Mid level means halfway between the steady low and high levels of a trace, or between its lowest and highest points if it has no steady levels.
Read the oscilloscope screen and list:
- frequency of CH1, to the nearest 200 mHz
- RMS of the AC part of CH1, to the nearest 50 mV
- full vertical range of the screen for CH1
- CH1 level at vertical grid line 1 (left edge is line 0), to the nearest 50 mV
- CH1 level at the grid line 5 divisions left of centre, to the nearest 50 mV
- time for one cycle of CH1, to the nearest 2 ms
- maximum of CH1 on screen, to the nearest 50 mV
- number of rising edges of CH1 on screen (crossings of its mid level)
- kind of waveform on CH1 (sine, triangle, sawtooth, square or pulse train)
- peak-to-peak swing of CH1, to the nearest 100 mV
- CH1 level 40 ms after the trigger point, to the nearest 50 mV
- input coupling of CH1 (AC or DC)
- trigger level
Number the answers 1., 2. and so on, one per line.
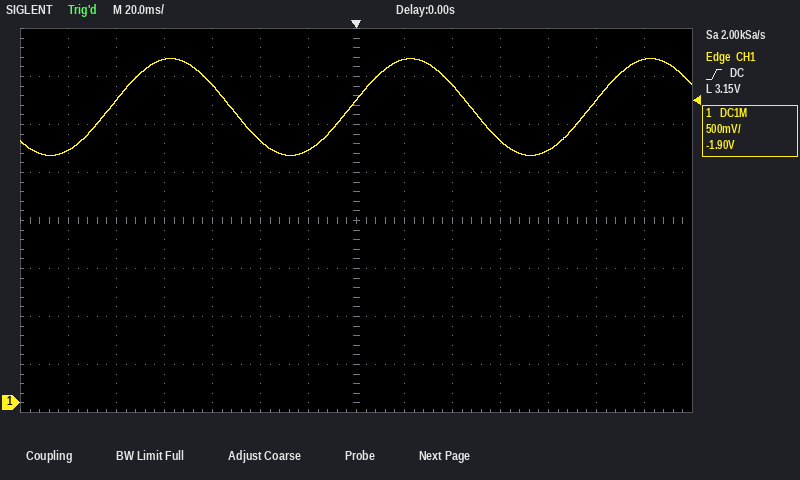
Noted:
1. 10.0 Hz
2. 350 mV
3. 4 V
4. 2.65 V
5. 3.15 V
6. 100 ms
7. 3.60 V
8. 3
9. sine
10. 1.00 V
11. 3.30 V
12. DC
13. 3.15 V
